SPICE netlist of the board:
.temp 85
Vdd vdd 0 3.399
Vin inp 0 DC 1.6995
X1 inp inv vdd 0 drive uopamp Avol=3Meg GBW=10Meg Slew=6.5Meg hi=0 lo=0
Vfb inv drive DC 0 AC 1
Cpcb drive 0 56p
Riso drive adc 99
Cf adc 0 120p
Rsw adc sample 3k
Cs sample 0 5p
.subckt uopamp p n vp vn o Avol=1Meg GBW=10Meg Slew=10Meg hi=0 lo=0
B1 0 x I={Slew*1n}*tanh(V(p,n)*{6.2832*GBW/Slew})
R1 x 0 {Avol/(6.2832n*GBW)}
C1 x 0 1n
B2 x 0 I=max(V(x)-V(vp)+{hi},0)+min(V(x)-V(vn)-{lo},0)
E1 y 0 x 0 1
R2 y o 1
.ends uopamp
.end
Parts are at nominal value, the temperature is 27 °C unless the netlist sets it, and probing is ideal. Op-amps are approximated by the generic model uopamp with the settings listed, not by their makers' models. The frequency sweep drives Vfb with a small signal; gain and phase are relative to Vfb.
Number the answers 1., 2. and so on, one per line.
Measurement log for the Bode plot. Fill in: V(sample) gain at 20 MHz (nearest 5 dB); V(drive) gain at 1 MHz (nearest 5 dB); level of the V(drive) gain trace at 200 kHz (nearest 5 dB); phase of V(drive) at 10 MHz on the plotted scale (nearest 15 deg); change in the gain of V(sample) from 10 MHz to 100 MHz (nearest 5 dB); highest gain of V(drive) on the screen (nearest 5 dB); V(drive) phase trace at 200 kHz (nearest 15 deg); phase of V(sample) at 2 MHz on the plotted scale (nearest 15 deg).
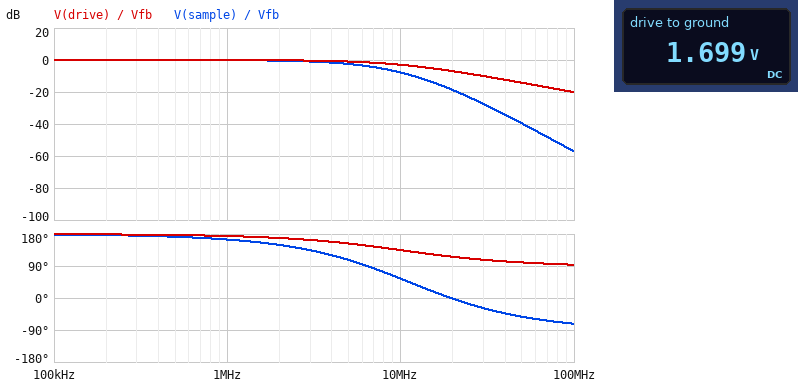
1. -20 dB
2. 0 dB
3. 0 dB
4. 135 deg
5. -50 dB
6. 0 dB
7. 180 deg
8. 150 deg
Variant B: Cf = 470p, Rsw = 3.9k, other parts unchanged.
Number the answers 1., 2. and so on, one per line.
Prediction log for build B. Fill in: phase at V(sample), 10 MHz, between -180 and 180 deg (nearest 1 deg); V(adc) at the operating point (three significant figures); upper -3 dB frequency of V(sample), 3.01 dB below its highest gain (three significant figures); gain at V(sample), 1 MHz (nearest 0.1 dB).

1. 13 deg
2. 1.70 V
3. 2.76 MHz
4. -0.5 dB
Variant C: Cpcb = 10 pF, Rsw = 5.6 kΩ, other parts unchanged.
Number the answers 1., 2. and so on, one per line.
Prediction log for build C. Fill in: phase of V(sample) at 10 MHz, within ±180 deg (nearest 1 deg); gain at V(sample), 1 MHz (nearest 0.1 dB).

1. 38 deg
2. -0.2 dB
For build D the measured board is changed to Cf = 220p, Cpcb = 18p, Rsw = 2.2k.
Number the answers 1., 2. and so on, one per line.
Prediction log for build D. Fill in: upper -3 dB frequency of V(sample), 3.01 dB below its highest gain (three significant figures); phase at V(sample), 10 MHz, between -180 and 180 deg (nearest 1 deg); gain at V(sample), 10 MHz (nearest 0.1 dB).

1. 4.83 MHz
2. 46 deg
3. -9.4 dB
